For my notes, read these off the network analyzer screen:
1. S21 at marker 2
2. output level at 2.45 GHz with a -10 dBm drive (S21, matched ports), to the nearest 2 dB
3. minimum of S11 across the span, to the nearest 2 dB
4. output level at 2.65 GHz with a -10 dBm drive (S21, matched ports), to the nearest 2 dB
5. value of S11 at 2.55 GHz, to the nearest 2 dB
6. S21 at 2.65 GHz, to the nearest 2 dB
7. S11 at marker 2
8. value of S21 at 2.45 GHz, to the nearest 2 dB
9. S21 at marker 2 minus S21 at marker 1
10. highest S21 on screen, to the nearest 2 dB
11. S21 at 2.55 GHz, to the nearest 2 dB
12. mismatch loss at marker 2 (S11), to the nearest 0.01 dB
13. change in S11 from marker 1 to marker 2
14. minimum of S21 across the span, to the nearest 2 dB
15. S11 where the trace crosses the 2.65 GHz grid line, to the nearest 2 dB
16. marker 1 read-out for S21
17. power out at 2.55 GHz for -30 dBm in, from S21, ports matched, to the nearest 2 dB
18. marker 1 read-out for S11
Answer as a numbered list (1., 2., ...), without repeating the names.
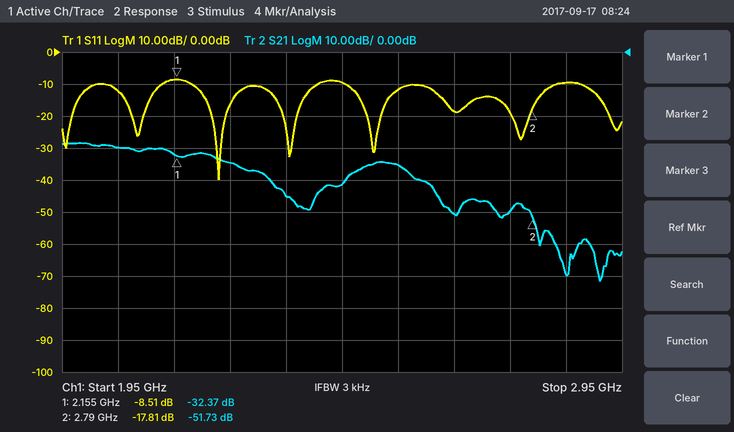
1. -51.73 dB
2. -52 dBm
3. -40 dB
4. -60 dBm
5. -12 dB
6. -50 dB
7. -17.81 dB
8. -42 dB
9. -19.36 dB
10. -28 dB
11. -36 dB
12. 0.07 dB
13. -9.30 dB
14. -72 dB
15. -18 dB
16. -32.37 dB
17. -66 dBm
18. -8.51 dB
